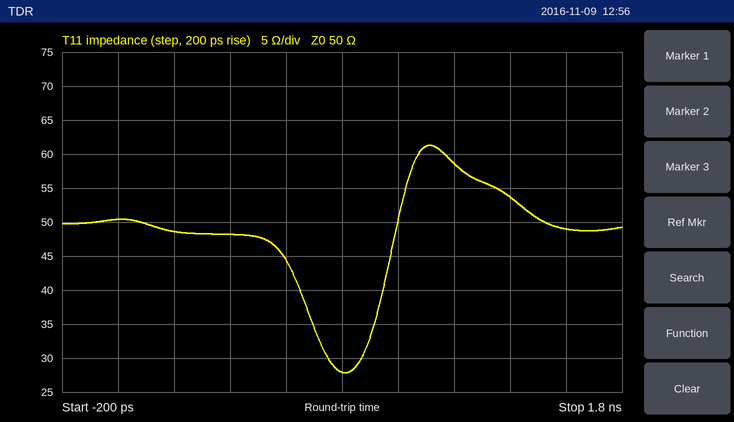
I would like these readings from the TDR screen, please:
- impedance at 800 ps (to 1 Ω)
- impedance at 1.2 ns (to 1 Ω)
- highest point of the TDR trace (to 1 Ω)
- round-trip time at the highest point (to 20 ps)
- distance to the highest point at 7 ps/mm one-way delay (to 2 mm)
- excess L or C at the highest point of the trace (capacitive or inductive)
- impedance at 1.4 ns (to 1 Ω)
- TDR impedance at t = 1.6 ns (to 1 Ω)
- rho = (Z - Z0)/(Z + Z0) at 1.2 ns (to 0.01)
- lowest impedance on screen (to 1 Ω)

28 Ω
59 Ω
61 Ω
1.12 ns
80 mm
inductive
54 Ω
49 Ω
+0.08
28 Ω
